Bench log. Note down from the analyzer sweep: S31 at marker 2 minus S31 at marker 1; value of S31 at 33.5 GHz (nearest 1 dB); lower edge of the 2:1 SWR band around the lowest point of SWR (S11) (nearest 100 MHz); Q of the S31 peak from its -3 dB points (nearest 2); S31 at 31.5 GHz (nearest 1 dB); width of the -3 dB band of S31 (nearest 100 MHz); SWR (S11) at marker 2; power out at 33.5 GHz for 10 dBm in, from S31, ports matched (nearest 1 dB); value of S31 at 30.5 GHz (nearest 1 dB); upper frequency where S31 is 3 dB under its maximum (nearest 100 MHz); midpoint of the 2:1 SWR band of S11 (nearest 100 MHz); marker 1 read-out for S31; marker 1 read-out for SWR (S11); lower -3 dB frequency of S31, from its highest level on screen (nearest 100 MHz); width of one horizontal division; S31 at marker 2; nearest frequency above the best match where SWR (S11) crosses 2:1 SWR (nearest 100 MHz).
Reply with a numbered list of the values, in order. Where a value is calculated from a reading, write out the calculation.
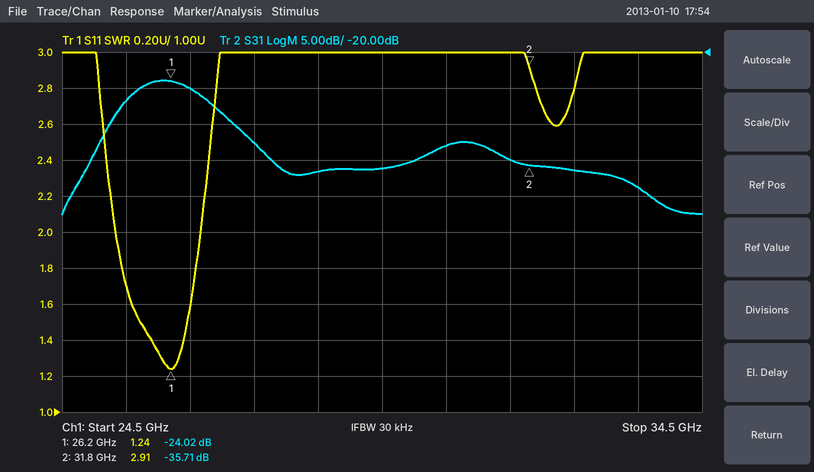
1. -35.71 − (-24.02) = -11.69 dB
2. -39 dB
3. 25.3 GHz
4. 26.15 GHz / 1.3 GHz ≈ 20
5. -35 dB
6. 26.8 GHz − 25.5 GHz = 1.3 GHz
7. 2.91
8. 10 dBm + (-39 dB) = -29 dBm
9. -33 dB
10. 26.8 GHz
11. 26.0 GHz
12. -24.02 dB
13. 1.24
14. 25.5 GHz
15. 1 GHz
16. -35.71 dB
17. 26.7 GHz
